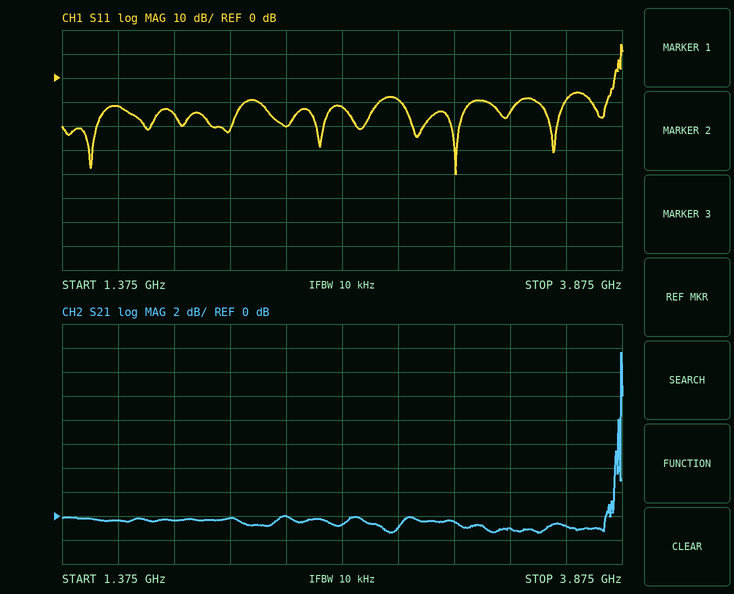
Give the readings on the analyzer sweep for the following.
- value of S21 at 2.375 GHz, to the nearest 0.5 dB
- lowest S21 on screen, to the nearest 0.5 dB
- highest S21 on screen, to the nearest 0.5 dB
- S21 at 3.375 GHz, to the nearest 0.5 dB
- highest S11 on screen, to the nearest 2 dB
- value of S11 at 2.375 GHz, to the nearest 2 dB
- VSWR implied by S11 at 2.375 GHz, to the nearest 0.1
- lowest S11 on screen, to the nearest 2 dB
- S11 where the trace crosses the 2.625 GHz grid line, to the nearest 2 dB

0.0 dB
-1.5 dB
13.5 dB
-1.0 dB
14 dB
-20 dB
1.2
-40 dB
-12 dB
